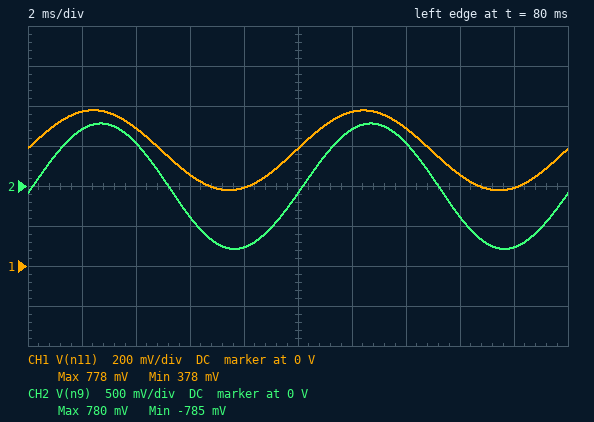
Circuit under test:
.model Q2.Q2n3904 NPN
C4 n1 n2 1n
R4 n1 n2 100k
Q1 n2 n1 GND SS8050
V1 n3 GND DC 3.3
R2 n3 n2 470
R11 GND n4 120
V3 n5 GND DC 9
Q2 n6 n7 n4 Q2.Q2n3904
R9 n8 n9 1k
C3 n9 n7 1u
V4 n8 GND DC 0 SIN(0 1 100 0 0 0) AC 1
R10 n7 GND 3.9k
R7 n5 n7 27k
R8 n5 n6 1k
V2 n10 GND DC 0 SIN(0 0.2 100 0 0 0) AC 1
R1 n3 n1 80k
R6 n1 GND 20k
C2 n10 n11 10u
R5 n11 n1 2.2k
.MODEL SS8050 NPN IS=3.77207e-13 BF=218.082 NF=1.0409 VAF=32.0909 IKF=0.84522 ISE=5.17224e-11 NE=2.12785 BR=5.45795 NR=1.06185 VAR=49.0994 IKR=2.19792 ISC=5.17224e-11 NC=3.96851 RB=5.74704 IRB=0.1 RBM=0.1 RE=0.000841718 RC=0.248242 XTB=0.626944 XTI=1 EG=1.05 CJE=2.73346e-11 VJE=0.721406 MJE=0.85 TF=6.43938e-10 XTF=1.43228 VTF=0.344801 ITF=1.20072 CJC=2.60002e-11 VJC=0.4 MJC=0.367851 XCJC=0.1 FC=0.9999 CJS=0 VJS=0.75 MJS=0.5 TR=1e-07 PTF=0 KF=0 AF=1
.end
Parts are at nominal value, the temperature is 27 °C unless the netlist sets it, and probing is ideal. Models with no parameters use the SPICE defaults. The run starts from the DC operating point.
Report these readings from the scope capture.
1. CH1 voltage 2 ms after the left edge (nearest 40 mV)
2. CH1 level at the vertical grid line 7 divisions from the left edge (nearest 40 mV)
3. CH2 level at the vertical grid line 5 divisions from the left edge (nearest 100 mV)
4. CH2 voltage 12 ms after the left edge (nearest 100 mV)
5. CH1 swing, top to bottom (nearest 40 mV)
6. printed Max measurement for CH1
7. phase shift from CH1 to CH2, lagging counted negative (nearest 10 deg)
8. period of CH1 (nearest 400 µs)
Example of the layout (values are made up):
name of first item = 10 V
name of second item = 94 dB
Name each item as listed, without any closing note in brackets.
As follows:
CH1 voltage 2 ms after the left edge = 760 mV
CH1 level at the vertical grid line 7 divisions from the left edge = 680 mV
CH2 level at the vertical grid line 5 divisions from the left edge = -100 mV
CH2 voltage 12 ms after the left edge = 700 mV
CH1 swing, top to bottom = 400 mV
printed Max measurement for CH1 = 778 mV
phase shift from CH1 to CH2, lagging counted negative = -10 deg
period of CH1 = 10.0 ms
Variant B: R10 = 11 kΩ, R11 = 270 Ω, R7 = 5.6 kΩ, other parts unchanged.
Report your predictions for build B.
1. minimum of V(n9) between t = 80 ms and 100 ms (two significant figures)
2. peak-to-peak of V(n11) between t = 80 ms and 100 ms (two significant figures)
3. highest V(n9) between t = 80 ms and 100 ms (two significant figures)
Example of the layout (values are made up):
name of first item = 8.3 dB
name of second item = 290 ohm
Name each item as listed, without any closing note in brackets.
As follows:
minimum of V(n9) between t = 80 ms and 100 ms = -800 mV
peak-to-peak of V(n11) between t = 80 ms and 100 ms = 400 mV
highest V(n9) between t = 80 ms and 100 ms = 800 mV
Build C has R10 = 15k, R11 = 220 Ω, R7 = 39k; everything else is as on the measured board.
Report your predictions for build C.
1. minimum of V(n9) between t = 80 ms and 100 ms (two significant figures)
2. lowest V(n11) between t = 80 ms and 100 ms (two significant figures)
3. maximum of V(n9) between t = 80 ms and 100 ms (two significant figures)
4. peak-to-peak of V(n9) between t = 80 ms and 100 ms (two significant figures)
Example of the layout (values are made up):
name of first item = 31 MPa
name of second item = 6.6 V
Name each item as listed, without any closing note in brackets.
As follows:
minimum of V(n9) between t = 80 ms and 100 ms = -870 mV
lowest V(n11) between t = 80 ms and 100 ms = 380 mV
maximum of V(n9) between t = 80 ms and 100 ms = 860 mV
peak-to-peak of V(n9) between t = 80 ms and 100 ms = 1.7 V
